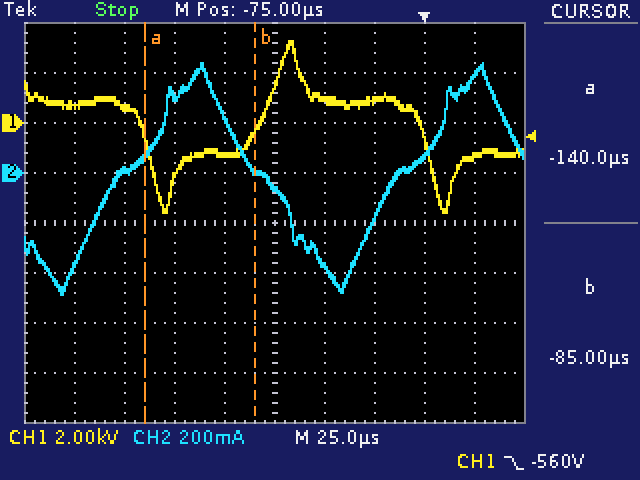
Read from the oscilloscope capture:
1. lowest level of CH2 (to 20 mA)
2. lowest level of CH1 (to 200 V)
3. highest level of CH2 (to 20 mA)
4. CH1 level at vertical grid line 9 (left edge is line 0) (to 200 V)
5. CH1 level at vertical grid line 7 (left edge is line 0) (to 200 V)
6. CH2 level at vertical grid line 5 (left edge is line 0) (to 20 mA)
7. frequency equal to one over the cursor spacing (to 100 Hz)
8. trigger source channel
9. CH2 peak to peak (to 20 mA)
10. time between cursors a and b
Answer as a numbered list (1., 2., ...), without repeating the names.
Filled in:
1. -480 mA
2. -3.6 kV
3. 440 mA
4. -1.4 kV
5. 800 V
6. -60 mA
7. 18.2 kHz
8. CH1
9. 920 mA
10. 55.0 µs
